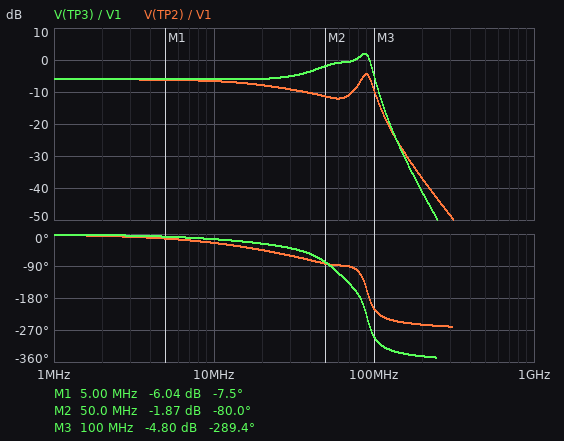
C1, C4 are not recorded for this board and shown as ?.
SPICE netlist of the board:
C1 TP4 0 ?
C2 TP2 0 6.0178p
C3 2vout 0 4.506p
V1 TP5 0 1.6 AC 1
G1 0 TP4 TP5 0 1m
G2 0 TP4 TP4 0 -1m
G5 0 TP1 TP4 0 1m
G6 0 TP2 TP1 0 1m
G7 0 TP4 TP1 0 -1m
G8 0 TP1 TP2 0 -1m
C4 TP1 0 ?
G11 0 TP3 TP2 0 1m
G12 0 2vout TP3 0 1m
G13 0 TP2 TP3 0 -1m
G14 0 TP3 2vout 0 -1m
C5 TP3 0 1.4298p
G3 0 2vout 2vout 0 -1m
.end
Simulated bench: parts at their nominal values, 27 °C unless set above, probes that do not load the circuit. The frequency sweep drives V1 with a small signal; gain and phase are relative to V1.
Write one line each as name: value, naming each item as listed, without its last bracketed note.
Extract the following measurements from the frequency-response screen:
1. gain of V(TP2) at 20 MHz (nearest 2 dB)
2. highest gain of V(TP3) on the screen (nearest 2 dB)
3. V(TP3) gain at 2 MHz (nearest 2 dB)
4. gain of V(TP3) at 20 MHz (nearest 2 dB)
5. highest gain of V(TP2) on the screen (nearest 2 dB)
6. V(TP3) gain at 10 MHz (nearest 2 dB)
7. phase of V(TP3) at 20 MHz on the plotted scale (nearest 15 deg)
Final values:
gain of V(TP2) at 20 MHz: -8 dB
highest gain of V(TP3) on the screen: 2 dB
V(TP3) gain at 2 MHz: -6 dB
gain of V(TP3) at 20 MHz: -6 dB
highest gain of V(TP2) on the screen: -4 dB
V(TP3) gain at 10 MHz: -6 dB
phase of V(TP3) at 20 MHz on the plotted scale: -30 deg
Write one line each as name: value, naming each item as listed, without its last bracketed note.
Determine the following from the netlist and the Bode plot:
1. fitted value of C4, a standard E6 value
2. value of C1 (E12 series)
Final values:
fitted value of C4, a standard E6 value: 2.2 pF
value of C1: 3.3 pF
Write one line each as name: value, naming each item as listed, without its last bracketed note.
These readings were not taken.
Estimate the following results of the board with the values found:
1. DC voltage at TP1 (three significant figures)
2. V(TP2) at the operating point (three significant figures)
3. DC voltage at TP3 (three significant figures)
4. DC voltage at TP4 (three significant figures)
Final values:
DC voltage at TP1: 800 mV
V(TP2) at the operating point: 800 mV
DC voltage at TP3: 800 mV
DC voltage at TP4: 800 mV
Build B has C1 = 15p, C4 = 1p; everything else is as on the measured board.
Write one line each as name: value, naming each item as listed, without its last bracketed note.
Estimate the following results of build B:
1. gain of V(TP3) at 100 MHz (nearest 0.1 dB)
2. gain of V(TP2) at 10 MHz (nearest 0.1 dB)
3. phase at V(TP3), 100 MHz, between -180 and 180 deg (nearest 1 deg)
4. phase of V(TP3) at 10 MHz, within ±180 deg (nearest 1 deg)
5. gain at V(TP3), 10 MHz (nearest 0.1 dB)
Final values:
gain of V(TP3) at 100 MHz: -1.8 dB
gain of V(TP2) at 10 MHz: -7.9 dB
phase at V(TP3), 100 MHz, between -180 and 180 deg: 76 deg
phase of V(TP3) at 10 MHz, within ±180 deg: -28 deg
gain at V(TP3), 10 MHz: -7.4 dB
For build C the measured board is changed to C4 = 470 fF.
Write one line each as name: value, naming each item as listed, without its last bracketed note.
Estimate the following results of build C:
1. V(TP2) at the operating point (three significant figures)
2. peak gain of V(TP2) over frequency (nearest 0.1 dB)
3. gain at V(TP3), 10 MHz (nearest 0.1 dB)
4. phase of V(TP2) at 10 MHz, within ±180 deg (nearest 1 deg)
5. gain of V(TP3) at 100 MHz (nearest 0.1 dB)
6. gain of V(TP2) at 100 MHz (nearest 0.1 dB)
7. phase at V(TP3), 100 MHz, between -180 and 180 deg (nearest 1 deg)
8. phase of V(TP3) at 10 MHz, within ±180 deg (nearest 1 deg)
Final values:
V(TP2) at the operating point: 800 mV
peak gain of V(TP2) over frequency: -3.7 dB
gain at V(TP3), 10 MHz: -6.2 dB
phase of V(TP2) at 10 MHz, within ±180 deg: -22 deg
gain of V(TP3) at 100 MHz: -5.1 dB
gain of V(TP2) at 100 MHz: -9.6 dB
phase at V(TP3), 100 MHz, between -180 and 180 deg: -160 deg
phase of V(TP3) at 10 MHz, within ±180 deg: -11 deg
